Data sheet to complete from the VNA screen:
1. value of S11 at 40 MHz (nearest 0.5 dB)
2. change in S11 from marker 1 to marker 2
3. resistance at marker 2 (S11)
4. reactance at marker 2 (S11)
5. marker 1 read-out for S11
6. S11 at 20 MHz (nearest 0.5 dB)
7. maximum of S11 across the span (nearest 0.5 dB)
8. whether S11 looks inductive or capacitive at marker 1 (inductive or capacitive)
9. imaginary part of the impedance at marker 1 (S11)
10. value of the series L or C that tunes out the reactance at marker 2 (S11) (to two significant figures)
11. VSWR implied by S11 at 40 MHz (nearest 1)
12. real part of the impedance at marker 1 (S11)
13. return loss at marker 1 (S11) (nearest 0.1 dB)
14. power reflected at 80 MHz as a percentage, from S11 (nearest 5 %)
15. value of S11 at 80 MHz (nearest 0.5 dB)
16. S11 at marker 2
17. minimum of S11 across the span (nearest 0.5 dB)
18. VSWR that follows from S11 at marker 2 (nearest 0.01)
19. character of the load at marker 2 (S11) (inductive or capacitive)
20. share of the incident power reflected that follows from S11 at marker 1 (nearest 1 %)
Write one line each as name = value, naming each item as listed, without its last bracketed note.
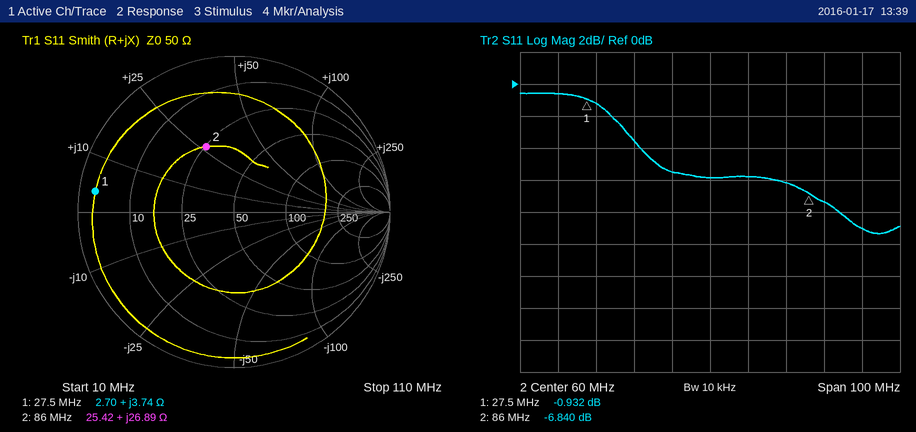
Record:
value of S11 at 40 MHz = -3.5 dB
change in S11 from marker 1 to marker 2 = -5.908 dB
resistance at marker 2 = 25.42 Ω
reactance at marker 2 = +26.89 Ω
marker 1 read-out for S11 = -0.932 dB
S11 at 20 MHz = -0.5 dB
maximum of S11 across the span = -0.5 dB
whether S11 looks inductive or capacitive at marker 1 = inductive
imaginary part of the impedance at marker 1 = +3.74 Ω
value of the series L or C that tunes out the reactance at marker 2 (S11) = 69 pF
VSWR implied by S11 at 40 MHz = 5
real part of the impedance at marker 1 = 2.70 Ω
return loss at marker 1 (S11) = 0.9 dB
power reflected at 80 MHz as a percentage, from S11 = 25 %
value of S11 at 80 MHz = -6.0 dB
S11 at marker 2 = -6.840 dB
minimum of S11 across the span = -9.5 dB
VSWR that follows from S11 at marker 2 = 2.67
character of the load at marker 2 (S11) = inductive
share of the incident power reflected that follows from S11 at marker 1 = 81 %
